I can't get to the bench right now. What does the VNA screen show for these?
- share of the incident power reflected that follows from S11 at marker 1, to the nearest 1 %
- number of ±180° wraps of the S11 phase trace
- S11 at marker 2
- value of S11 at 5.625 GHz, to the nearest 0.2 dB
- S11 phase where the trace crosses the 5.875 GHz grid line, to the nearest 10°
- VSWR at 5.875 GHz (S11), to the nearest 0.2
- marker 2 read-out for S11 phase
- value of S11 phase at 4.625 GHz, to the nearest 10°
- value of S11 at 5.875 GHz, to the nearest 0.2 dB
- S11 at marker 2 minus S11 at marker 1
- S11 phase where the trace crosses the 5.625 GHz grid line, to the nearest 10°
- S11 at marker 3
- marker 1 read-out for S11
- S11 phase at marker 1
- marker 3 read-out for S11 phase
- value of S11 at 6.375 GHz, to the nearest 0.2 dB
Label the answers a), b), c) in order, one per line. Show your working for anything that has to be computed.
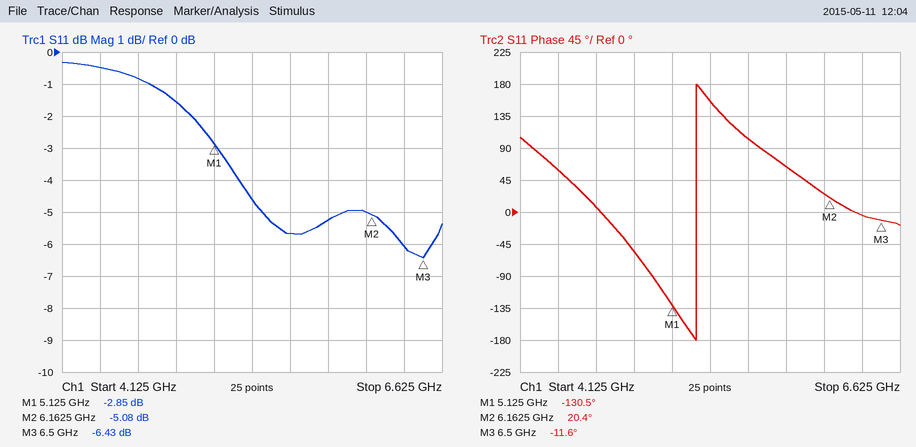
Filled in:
a) 10^(-2.85/10) ≈ 52 %
b) 1
c) -5.08 dB
d) -5.6 dB
e) 60°
f) |Γ| = 10^(-5.2/20) = 0.5495; VSWR = (1 + 0.5495)/(1 − 0.5495) ≈ 3.4
g) 20.4°
h) 10°
i) -5.2 dB
j) -5.08 − (-2.85) = -2.23 dB
k) 100°
l) -6.43 dB
m) -2.85 dB
n) -130.5°
o) -11.6°
p) -6.0 dB
